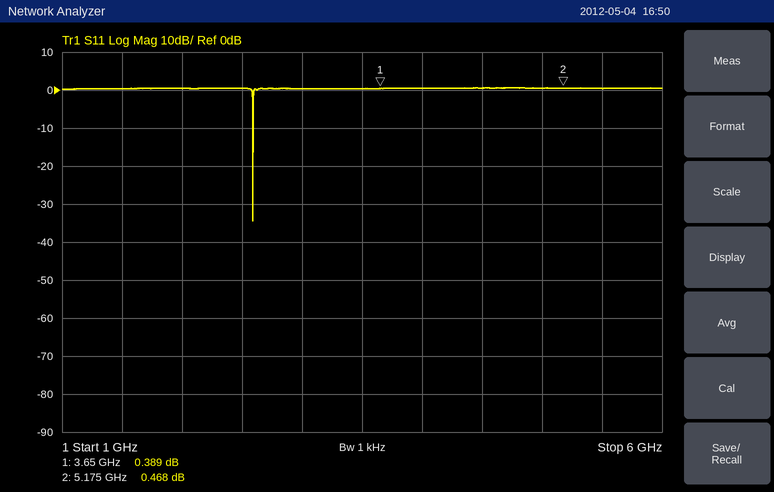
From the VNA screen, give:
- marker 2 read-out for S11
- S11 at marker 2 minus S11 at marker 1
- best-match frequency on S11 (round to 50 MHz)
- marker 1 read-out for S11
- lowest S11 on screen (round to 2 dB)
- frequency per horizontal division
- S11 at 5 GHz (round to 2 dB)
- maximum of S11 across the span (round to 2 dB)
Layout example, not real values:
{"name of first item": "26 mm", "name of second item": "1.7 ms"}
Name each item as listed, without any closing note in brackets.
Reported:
{"marker 2 read-out for S11": "0.468 dB", "S11 at marker 2 minus S11 at marker 1": "0.079 dB", "best-match frequency on S11": "2.60 GHz", "marker 1 read-out for S11": "0.389 dB", "lowest S11 on screen": "-34 dB", "frequency per horizontal division": "500 MHz", "S11 at 5 GHz": "0 dB", "maximum of S11 across the span": "0 dB"}
